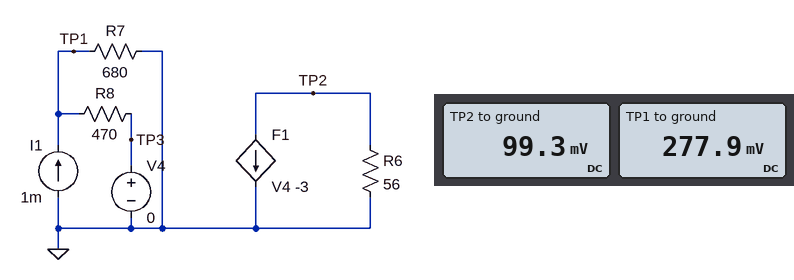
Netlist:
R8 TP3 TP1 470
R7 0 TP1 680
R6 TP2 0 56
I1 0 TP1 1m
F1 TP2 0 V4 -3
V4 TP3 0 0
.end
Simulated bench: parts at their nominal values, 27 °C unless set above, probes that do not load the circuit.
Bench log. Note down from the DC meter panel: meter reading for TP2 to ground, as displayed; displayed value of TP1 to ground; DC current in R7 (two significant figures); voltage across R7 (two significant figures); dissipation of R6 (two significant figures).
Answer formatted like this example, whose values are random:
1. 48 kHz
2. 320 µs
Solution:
1. 99.3 mV
2. 277.9 mV
3. 410 µA
4. 280 mV
5. 180 µW
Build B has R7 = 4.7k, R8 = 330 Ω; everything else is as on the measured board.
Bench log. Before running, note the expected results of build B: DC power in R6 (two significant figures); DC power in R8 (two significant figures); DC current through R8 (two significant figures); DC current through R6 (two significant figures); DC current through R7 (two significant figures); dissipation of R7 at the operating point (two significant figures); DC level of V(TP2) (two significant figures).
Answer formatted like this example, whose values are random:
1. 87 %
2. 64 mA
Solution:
1. 440 µW
2. 290 µW
3. 930 µA
4. 2.8 mA
5. 66 µA
6. 20 µW
7. 160 mV
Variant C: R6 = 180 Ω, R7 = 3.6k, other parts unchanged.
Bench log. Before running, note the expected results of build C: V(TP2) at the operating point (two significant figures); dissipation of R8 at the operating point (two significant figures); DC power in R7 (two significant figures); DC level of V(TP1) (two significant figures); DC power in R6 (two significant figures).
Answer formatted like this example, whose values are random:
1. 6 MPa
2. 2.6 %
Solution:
1. 480 mV
2. 370 µW
3. 48 µW
4. 420 mV
5. 1.3 mW
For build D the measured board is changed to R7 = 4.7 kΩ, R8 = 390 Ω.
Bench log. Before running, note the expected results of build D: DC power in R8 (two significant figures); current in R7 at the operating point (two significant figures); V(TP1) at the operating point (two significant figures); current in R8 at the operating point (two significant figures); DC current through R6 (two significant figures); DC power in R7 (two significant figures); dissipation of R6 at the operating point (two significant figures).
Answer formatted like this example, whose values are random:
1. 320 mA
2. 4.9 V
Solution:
1. 330 µW
2. 77 µA
3. 360 mV
4. 920 µA
5. 2.8 mA
6. 28 µW
7. 430 µW
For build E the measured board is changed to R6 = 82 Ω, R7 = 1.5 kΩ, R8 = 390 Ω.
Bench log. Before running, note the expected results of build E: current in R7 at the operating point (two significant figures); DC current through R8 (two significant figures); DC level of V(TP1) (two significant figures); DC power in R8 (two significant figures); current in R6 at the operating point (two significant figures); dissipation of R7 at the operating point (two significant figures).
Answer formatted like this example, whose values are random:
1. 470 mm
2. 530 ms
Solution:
1. 210 µA
2. 790 µA
3. 310 mV
4. 250 µW
5. 2.4 mA
6. 64 µW
